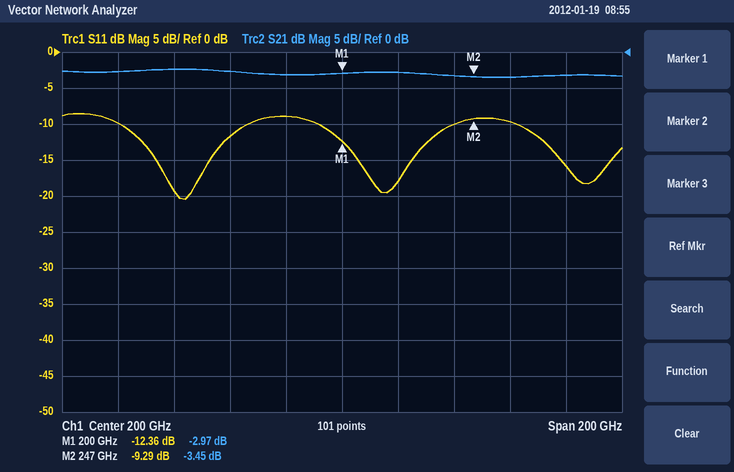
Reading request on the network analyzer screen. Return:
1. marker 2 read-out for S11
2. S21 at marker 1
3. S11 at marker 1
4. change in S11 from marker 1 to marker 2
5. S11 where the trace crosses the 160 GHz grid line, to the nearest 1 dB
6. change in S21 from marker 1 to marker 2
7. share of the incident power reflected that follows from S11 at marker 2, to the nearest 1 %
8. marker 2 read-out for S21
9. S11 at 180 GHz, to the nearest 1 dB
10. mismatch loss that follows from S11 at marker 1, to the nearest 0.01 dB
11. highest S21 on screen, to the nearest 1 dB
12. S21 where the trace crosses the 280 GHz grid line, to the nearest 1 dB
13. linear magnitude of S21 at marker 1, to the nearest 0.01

-9.29 dB
-2.97 dB
-12.36 dB
3.07 dB
-12 dB
-0.48 dB
12 %
-3.45 dB
-9 dB
0.26 dB
-2 dB
-3 dB
0.71
